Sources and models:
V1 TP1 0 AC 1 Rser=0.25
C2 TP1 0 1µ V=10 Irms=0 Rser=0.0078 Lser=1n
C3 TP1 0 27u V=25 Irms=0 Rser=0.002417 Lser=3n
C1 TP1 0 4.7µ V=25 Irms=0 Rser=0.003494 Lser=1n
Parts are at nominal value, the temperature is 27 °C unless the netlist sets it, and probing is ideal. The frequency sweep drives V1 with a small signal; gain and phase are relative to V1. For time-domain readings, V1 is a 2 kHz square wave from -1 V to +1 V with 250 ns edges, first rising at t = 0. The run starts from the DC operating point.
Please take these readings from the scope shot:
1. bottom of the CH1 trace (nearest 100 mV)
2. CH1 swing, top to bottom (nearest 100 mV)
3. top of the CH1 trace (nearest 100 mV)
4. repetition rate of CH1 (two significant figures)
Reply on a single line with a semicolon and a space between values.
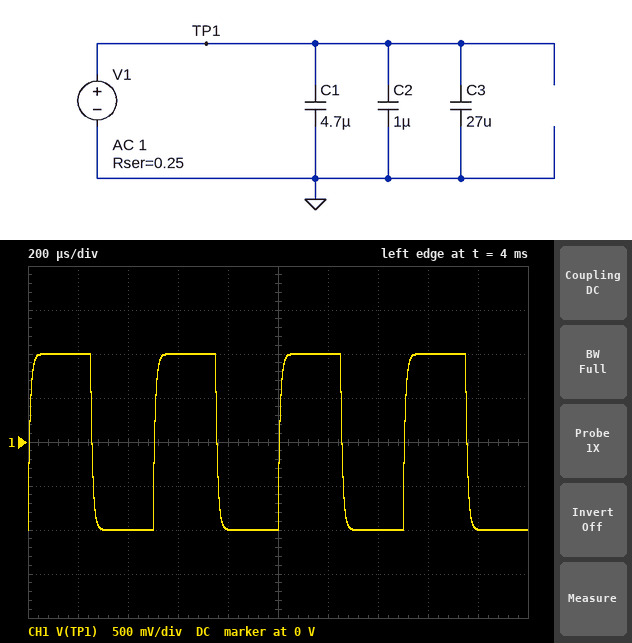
-1.0 V; 2.0 V; 1.0 V; 2.0 kHz
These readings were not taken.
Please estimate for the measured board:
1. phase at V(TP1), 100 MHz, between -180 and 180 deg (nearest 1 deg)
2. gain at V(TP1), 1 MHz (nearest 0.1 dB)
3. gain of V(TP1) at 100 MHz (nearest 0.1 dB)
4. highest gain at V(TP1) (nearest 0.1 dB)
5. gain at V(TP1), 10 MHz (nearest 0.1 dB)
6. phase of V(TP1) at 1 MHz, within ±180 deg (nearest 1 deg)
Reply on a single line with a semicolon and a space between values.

43 deg; -19.9 dB; -2.7 dB; 0 dB; -20.8 dB; 55 deg
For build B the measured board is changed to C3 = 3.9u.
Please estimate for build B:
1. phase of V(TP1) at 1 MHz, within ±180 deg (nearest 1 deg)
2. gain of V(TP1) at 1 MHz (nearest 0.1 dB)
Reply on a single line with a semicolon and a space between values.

-81 deg; -26.9 dB
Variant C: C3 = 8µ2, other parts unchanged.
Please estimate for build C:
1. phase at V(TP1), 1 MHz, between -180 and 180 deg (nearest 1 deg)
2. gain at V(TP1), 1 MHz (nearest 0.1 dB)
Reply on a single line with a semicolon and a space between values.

-18 deg; -40.5 dB
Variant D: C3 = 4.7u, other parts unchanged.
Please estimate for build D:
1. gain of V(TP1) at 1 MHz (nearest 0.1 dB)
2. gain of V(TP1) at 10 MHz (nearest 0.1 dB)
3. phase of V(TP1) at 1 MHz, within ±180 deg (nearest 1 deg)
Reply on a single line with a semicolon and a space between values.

-28.7 dB; -20.8 dB; -80 deg
